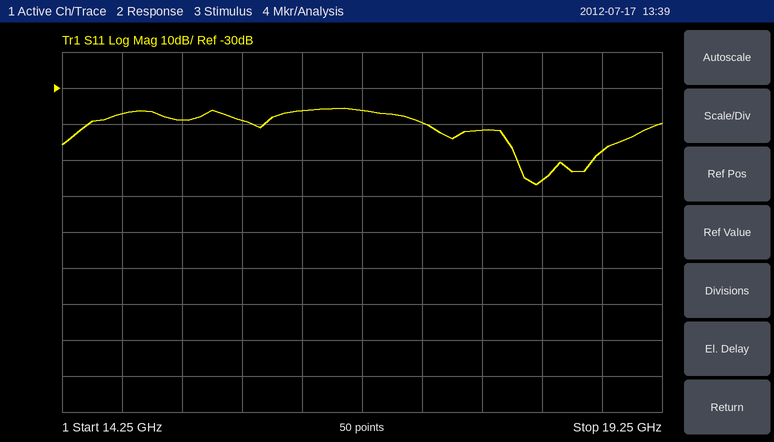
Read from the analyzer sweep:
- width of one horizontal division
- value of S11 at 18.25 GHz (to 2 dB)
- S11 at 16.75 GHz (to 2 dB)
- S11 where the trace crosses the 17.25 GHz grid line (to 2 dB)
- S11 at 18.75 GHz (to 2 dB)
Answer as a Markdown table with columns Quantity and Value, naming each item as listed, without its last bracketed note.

| Quantity | Value |
|---|---|
| width of one horizontal division | 500 MHz |
| value of S11 at 18.25 GHz | -56 dB |
| S11 at 16.75 GHz | -36 dB |
| S11 where the trace crosses the 17.25 GHz grid line | -40 dB |
| S11 at 18.75 GHz | -48 dB |
